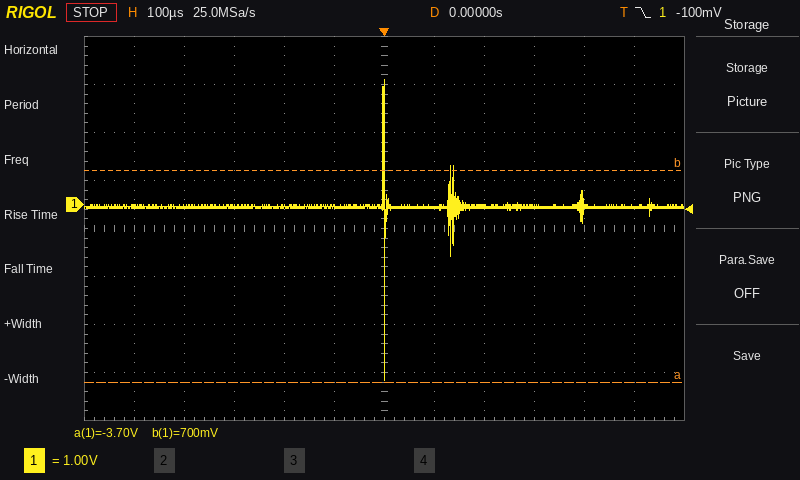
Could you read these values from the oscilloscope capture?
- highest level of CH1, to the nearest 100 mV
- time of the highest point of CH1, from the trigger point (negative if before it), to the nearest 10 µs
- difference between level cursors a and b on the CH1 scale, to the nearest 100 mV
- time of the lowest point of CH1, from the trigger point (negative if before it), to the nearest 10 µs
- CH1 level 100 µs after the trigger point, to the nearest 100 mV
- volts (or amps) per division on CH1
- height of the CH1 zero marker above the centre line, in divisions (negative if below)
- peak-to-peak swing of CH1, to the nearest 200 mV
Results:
2.6 V
0 µs
4.4 V
0 µs
-100 mV
1 V
+0.5 div
6.2 V
